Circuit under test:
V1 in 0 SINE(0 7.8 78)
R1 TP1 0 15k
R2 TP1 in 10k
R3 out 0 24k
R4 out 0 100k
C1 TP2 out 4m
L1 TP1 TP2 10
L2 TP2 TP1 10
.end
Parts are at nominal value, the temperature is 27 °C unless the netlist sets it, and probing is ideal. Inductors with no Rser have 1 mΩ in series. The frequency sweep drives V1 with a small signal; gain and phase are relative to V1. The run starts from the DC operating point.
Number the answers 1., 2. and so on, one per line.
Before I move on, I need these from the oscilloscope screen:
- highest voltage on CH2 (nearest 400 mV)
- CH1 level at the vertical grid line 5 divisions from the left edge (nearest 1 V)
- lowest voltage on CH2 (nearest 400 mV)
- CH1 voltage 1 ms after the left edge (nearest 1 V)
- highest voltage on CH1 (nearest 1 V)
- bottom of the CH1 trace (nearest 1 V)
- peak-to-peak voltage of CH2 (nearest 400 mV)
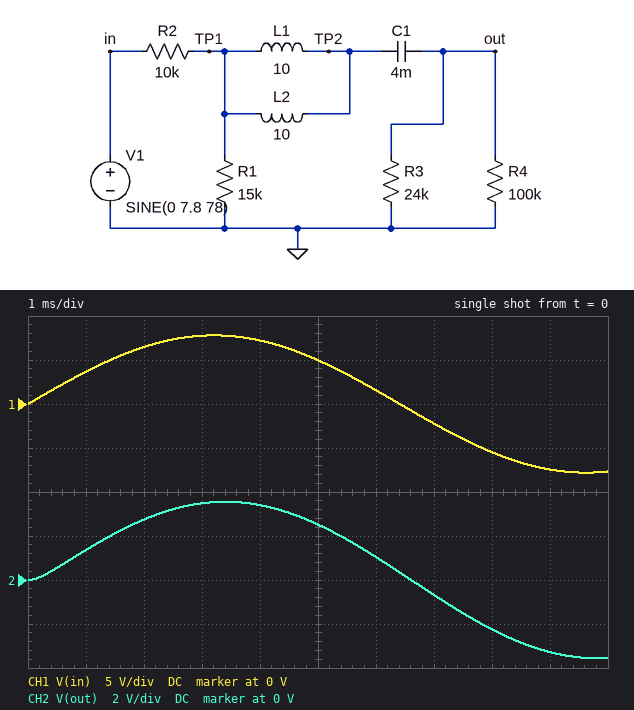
1. 3.6 V
2. 5 V
3. -3.6 V
4. 4 V
5. 8 V
6. -8 V
7. 7.2 V
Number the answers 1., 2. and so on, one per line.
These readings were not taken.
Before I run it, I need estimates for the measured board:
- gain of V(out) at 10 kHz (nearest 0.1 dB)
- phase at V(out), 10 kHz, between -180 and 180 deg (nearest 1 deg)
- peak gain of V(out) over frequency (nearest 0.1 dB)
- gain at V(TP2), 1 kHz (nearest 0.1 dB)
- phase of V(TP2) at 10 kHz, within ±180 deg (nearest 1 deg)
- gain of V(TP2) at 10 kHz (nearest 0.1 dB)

1. -28.7 dB
2. -85 deg
3. -6.8 dB
4. -10.8 dB
5. -85 deg
6. -28.7 dB
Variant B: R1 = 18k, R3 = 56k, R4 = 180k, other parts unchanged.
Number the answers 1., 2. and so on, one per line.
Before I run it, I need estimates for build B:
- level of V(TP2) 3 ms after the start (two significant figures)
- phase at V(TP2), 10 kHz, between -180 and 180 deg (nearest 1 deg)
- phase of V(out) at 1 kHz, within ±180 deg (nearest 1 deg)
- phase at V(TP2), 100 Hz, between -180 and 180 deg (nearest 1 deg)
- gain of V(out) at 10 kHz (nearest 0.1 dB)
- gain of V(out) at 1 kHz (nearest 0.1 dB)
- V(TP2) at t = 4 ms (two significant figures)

1. 4.3 V
2. -81 deg
3. -33 deg
4. -4 deg
5. -21.3 dB
6. -6.5 dB
7. 4.1 V
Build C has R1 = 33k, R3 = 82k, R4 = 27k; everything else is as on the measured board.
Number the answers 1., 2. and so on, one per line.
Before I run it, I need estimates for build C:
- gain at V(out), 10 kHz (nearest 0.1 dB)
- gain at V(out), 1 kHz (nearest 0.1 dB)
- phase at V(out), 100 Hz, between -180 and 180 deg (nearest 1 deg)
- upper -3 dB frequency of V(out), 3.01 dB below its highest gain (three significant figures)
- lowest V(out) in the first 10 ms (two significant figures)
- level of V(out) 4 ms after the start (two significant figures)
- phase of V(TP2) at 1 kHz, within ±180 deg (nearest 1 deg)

1. -26.1 dB
2. -8.6 dB
3. -6 deg
4. 891 Hz
5. -4.3 V
6. 4.1 V
7. -48 deg
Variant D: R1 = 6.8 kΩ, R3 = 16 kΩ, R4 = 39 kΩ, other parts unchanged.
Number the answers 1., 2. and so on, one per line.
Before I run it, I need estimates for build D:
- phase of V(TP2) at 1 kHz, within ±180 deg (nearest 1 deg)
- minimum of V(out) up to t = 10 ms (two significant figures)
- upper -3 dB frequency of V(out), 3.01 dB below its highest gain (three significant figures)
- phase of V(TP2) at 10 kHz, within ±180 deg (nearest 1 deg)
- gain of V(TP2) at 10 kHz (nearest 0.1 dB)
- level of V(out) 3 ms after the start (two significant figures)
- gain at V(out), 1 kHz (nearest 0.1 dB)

1. -64 deg
2. -2.3 V
3. 490 Hz
4. -87 deg
5. -36.7 dB
6. 2.2 V
7. -17.6 dB
